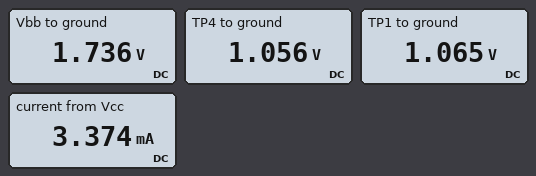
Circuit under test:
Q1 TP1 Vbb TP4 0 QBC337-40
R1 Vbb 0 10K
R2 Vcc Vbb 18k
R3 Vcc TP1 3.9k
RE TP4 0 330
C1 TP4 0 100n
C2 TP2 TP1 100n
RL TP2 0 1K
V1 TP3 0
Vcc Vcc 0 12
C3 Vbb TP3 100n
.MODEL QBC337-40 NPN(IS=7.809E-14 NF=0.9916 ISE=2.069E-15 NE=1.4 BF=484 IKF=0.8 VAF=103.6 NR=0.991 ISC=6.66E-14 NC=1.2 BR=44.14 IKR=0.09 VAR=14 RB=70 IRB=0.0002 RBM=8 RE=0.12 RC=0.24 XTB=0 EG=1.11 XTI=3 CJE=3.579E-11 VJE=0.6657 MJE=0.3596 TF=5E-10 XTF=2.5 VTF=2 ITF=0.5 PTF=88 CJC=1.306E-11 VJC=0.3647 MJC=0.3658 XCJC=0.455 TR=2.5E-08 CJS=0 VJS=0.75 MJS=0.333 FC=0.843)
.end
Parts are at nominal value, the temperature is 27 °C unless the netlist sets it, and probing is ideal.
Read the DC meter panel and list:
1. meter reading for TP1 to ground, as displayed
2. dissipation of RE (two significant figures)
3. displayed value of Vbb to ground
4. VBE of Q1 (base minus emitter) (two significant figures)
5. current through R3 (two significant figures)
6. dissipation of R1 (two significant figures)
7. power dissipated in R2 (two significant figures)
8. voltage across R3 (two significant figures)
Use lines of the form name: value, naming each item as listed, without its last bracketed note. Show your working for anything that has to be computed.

meter reading for TP1 to ground, as displayed: 1.065 V
dissipation of RE: (1.056 V)^2 / 330 Ω = 3.4 mW
displayed value of Vbb to ground: 1.736 V
VBE of Q1 (base minus emitter): 1.736 V - 1.056 V = 680 mV
current through R3: (12 V - 1.065 V) / 3.9 kΩ = 2.8 mA
dissipation of R1: (1.736 V)^2 / 10 kΩ = 300 µW
power dissipated in R2: (12 V - 1.736 V)^2 / 18 kΩ = 5.9 mW
voltage across R3: 12 V - 1.065 V = 11 V
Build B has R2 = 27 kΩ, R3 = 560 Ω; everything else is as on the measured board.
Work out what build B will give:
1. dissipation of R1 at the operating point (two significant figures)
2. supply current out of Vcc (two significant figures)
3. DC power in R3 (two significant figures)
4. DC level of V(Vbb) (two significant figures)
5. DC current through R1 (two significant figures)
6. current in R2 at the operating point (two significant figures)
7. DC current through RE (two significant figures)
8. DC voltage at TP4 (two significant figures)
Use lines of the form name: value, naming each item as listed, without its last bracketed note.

dissipation of R1 at the operating point: 980 µW
supply current out of Vcc: 7.8 mA
DC power in R3: 31 mW
DC level of V(Vbb): 3.1 V
DC current through R1: 310 µA
current in R2 at the operating point: 330 µA
DC current through RE: 7.5 mA
DC voltage at TP4: 2.5 V
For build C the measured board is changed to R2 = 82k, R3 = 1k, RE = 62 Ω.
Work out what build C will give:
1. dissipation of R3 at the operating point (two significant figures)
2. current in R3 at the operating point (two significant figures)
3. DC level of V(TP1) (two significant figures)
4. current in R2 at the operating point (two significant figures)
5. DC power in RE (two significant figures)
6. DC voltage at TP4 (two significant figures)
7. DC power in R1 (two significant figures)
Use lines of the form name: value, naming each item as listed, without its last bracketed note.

dissipation of R3 at the operating point: 64 mW
current in R3 at the operating point: 8.0 mA
DC level of V(TP1): 4.0 V
current in R2 at the operating point: 130 µA
DC power in RE: 4.0 mW
DC voltage at TP4: 500 mV
DC power in R1: 130 µW
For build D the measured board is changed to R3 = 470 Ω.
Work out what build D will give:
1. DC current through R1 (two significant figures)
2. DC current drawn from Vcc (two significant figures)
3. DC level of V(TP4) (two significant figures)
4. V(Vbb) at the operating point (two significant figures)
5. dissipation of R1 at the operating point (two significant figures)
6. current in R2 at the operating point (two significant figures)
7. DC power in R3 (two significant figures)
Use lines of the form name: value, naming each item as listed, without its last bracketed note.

DC current through R1: 410 µA
DC current drawn from Vcc: 11 mA
DC level of V(TP4): 3.5 V
V(Vbb) at the operating point: 4.1 V
dissipation of R1 at the operating point: 1.7 mW
current in R2 at the operating point: 440 µA
DC power in R3: 52 mW
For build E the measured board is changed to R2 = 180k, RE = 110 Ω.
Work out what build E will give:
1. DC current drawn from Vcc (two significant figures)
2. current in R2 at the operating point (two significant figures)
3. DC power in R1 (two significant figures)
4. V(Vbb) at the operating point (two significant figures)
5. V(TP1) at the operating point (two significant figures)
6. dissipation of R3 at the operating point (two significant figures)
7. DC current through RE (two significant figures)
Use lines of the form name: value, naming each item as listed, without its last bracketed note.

DC current drawn from Vcc: 500 µA
current in R2 at the operating point: 63 µA
DC power in R1: 39 µW
V(Vbb) at the operating point: 620 mV
V(TP1) at the operating point: 10 V
dissipation of R3 at the operating point: 760 µW
DC current through RE: 440 µA
